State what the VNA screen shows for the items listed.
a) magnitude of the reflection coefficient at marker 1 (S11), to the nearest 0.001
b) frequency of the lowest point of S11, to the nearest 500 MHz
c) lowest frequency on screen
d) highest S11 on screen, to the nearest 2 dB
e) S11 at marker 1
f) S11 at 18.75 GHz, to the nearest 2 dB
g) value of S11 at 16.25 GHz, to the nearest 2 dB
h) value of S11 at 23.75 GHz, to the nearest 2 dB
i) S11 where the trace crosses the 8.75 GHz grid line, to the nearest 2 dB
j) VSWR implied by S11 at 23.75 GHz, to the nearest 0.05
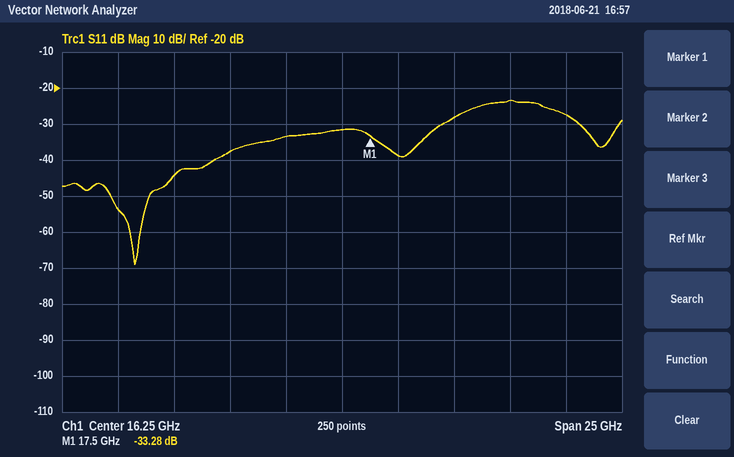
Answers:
0.022
7.0 GHz
3.75 GHz
-24 dB
-33.28 dB
-38 dB
-32 dB
-24 dB
-44 dB
1.15
